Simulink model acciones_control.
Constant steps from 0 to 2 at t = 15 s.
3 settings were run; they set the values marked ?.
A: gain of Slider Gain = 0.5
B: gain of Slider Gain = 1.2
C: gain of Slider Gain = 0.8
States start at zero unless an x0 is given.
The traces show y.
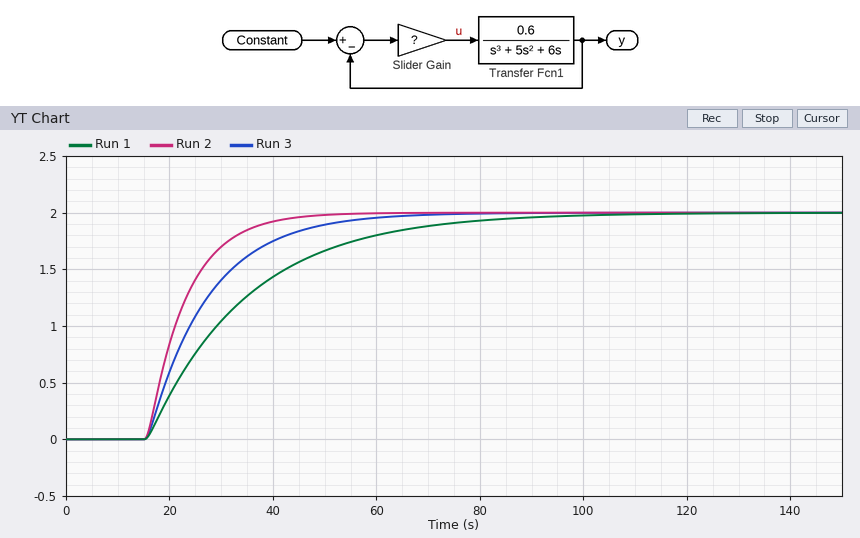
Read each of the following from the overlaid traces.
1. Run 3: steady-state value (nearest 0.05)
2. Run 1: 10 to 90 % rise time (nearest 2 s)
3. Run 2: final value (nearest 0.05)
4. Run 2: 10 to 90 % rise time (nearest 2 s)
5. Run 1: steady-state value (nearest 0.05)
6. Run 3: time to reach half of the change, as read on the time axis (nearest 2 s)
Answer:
2.00
42 s
2.00
16 s
2.00
24 s
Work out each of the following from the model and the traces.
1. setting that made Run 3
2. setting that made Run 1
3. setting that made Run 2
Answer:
C
A
B
